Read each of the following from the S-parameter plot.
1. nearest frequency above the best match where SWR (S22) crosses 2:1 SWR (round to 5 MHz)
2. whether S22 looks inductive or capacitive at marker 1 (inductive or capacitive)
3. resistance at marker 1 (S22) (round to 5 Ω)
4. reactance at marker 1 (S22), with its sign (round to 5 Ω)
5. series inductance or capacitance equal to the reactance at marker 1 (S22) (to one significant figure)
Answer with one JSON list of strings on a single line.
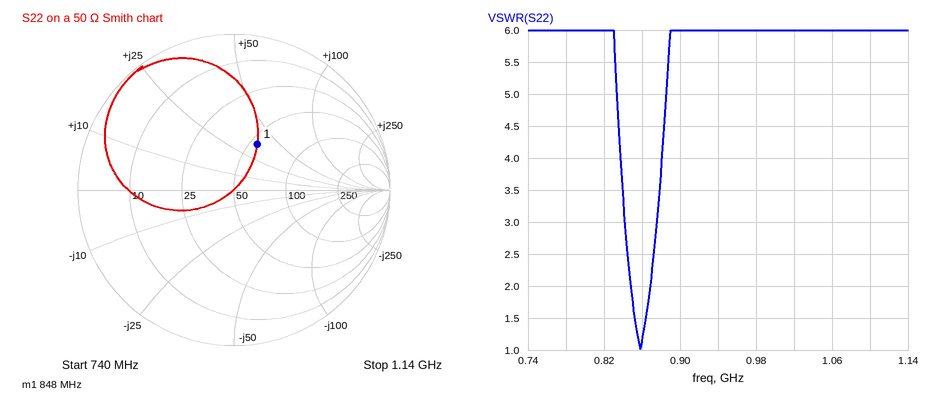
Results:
["870 MHz", "inductive", "55 Ω", "+35 Ω", "7 nH"]
